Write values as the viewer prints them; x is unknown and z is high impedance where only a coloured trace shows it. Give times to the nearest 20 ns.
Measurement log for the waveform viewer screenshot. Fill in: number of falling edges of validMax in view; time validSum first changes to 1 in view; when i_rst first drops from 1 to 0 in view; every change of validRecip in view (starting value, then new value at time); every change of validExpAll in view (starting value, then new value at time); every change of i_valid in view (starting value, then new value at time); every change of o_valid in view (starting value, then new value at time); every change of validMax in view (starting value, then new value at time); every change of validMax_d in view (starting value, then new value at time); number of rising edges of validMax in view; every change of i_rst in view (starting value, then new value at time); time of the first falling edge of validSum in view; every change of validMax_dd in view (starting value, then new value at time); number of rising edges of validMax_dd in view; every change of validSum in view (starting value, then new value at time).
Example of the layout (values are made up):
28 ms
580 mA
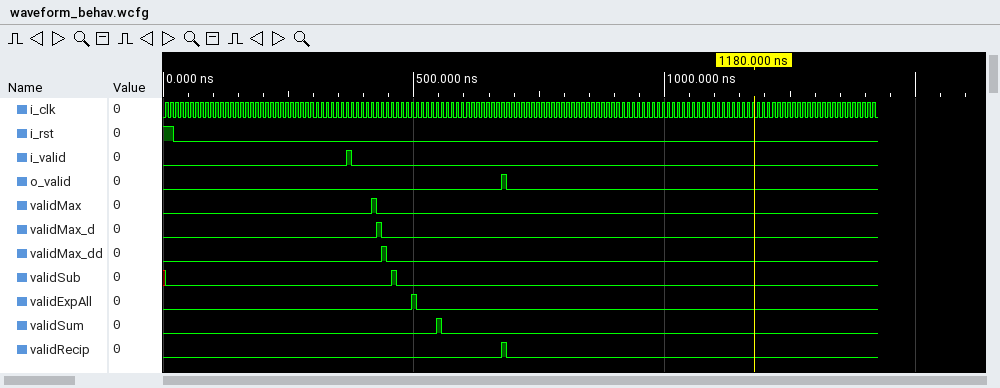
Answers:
1
540 ns
20 ns
0, 1 at 680 ns, 0 at 680 ns
0, 1 at 500 ns, 0 at 500 ns
0, 1 at 360 ns, 0 at 380 ns
0, 1 at 680 ns, 0 at 680 ns
0, 1 at 420 ns, 0 at 420 ns
0, 1 at 420 ns, 0 at 440 ns
1
1, 0 at 20 ns
560 ns
0, 1 at 440 ns, 0 at 440 ns
1
0, 1 at 540 ns, 0 at 560 ns
